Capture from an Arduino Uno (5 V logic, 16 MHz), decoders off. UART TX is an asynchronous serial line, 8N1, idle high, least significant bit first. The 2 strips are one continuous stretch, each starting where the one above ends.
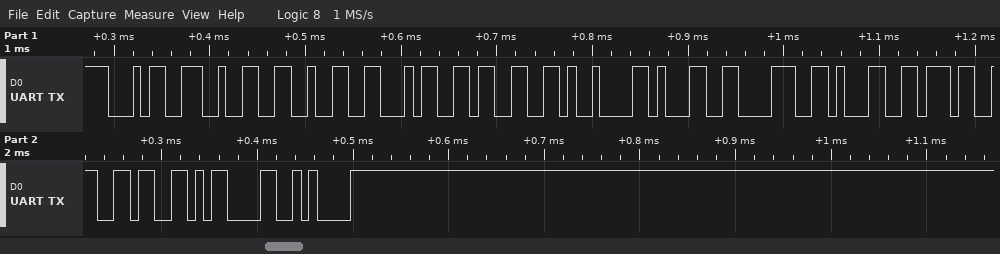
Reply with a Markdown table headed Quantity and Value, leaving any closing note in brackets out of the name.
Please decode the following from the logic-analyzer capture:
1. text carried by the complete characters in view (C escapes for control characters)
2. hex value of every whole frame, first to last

| Quantity | Value |
|---|---|
| text carried by the complete characters in view | "42243\t18176\r\n" |
| hex value of every whole frame, first to last | 34 32 32 34 33 09 31 38 31 37 36 0D 0A |
